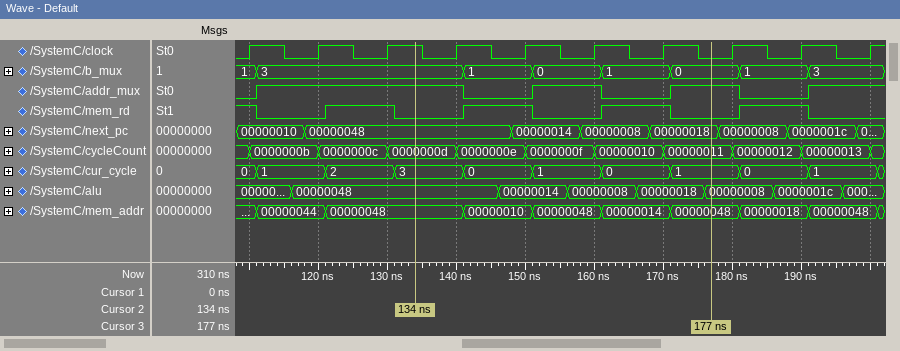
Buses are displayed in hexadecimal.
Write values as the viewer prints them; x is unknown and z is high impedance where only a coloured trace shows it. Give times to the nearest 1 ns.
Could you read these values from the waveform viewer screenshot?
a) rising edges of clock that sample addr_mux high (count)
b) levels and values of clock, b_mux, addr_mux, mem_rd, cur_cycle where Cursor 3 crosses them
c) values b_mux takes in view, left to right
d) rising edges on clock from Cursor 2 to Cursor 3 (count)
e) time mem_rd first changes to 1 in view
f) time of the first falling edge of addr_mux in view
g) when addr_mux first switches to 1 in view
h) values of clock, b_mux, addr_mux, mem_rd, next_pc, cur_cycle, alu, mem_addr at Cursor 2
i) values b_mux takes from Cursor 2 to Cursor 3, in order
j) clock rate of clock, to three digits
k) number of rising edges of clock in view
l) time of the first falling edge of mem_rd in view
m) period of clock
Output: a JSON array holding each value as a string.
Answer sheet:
["6", "clock=0, b_mux=0, addr_mux=1, mem_rd=0, cur_cycle=1", "1, 3, 1, 0, 1, 0, 1, 3", "4", "121 ns", "141 ns", "111 ns", "clock=1, b_mux=3, addr_mux=1, mem_rd=0, next_pc=00000048, cur_cycle=3, alu=00000048, mem_addr=00000048", "3, 1, 0, 1, 0", "100 MHz", "10", "111 ns", "10 ns"]
